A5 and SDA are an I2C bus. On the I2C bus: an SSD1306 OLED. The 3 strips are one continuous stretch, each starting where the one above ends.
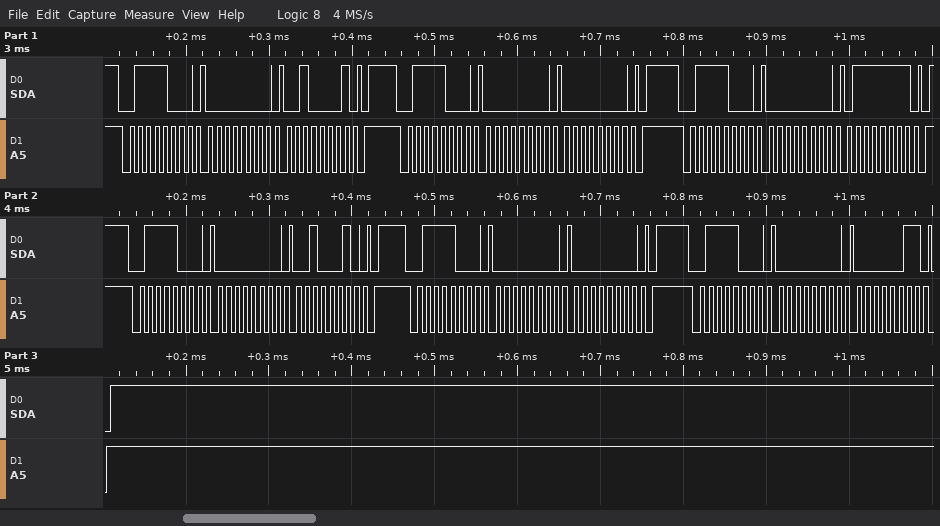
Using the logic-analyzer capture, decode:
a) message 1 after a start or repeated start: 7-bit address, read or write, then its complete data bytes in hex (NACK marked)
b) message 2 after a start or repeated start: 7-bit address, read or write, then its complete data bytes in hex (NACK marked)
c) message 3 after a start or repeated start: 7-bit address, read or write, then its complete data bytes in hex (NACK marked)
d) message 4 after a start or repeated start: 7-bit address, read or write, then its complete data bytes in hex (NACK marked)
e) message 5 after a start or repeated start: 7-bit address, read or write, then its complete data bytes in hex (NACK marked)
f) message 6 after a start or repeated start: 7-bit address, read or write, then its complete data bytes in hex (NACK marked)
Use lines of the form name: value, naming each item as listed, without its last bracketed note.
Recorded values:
message 1 after a start or repeated start: 7-bit address, read or write, then its complete data bytes in hex: 0x3C write: 00 21
message 2 after a start or repeated start: 7-bit address, read or write, then its complete data bytes in hex: 0x3C write: 00 00
message 3 after a start or repeated start: 7-bit address, read or write, then its complete data bytes in hex: 0x3C write: 00 7F
message 4 after a start or repeated start: 7-bit address, read or write, then its complete data bytes in hex: 0x3C write: 00 22
message 5 after a start or repeated start: 7-bit address, read or write, then its complete data bytes in hex: 0x3C write: 00 00
message 6 after a start or repeated start: 7-bit address, read or write, then its complete data bytes in hex: 0x3C write: 00 03
